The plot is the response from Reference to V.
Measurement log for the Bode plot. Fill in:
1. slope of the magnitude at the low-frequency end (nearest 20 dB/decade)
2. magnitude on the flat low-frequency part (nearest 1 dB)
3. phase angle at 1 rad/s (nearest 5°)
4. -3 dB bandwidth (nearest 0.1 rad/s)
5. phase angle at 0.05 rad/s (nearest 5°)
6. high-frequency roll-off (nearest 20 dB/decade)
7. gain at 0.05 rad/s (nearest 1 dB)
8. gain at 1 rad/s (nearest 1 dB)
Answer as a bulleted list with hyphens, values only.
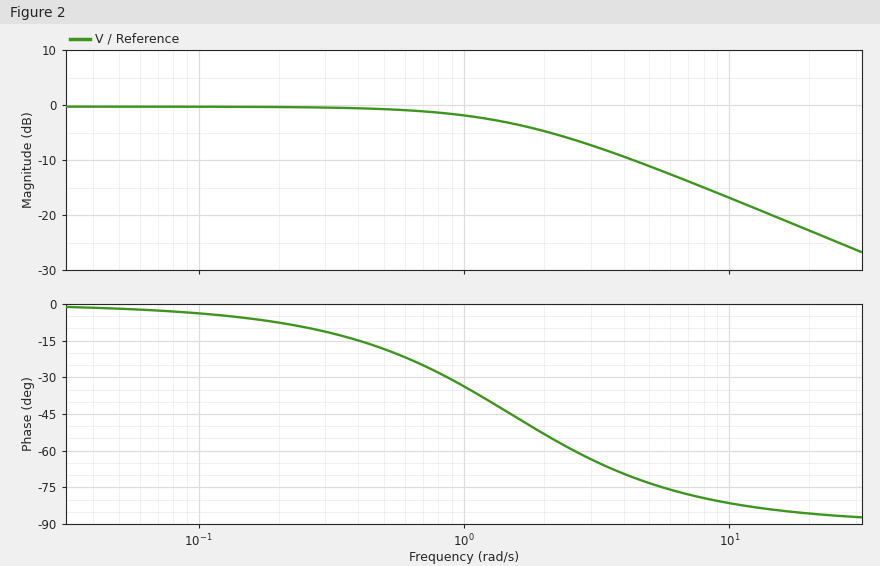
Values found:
- 0 dB/decade
- 0 dB
- -35°
- 1.5 rad/s
- 0°
- -20 dB/decade
- 0 dB
- -2 dB
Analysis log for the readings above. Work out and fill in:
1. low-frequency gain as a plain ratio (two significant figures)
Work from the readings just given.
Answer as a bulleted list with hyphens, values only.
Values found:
- 1.0
